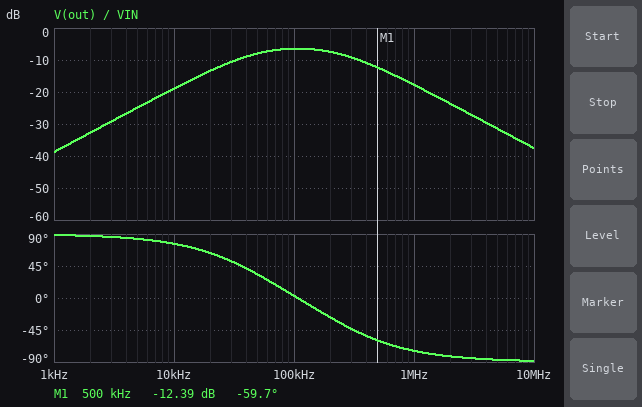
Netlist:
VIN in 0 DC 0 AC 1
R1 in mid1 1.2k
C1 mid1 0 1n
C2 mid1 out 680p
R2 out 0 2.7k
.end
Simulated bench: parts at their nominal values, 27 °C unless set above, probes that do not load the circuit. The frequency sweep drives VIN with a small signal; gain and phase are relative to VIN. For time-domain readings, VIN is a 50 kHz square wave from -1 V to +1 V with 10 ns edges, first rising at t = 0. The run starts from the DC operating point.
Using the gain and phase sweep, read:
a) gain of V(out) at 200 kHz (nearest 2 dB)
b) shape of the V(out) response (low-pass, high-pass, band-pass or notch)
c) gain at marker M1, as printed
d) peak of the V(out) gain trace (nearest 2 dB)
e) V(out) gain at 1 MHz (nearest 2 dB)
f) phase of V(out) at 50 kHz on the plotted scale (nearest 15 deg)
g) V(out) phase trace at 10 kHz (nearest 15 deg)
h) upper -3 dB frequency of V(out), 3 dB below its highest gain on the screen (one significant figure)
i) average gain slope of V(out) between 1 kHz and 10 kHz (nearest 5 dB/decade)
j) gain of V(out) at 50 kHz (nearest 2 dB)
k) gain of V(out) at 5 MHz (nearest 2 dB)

-8 dB
band-pass
-12.39 dB
-6 dB
-18 dB
30 deg
75 deg
300 kHz
20 dB/decade
-8 dB
-32 dB
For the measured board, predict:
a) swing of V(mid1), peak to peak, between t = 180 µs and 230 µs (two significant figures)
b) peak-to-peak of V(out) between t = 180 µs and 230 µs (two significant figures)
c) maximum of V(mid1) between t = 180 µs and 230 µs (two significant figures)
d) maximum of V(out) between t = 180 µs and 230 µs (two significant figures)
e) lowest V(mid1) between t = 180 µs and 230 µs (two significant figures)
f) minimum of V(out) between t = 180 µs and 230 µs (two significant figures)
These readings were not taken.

1.9 V
1.4 V
960 mV
720 mV
-960 mV
-720 mV
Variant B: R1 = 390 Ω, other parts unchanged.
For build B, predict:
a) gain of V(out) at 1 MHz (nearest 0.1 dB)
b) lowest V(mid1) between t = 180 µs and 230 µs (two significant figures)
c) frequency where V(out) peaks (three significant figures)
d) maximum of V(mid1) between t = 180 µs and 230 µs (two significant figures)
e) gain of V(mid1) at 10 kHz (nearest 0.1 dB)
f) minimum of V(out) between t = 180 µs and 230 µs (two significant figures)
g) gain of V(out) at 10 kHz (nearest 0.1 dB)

-8.7 dB
-1.0 V
188 kHz
1.0 V
0 dB
-1.2 V
-18.8 dB
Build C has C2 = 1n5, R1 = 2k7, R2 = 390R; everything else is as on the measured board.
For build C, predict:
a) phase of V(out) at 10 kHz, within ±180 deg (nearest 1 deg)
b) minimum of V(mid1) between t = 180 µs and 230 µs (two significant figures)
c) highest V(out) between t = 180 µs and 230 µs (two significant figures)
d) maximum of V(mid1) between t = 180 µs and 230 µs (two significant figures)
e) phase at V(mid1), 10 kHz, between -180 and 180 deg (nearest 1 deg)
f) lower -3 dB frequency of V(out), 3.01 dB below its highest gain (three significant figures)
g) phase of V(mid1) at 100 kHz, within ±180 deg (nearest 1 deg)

65 deg
-630 mV
120 mV
630 mV
-23 deg
21.1 kHz
-65 deg
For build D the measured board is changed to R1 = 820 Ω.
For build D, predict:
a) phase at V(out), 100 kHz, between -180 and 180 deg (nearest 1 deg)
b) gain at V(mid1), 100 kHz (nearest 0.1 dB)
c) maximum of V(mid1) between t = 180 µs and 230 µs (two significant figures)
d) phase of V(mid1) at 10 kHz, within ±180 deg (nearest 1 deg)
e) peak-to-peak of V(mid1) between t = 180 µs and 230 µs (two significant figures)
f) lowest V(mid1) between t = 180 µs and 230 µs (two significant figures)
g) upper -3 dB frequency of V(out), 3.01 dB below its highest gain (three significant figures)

11 deg
-2.6 dB
980 mV
-5 deg
2.0 V
-980 mV
384 kHz
